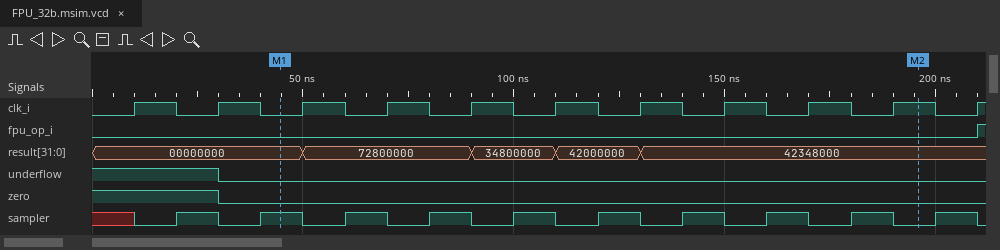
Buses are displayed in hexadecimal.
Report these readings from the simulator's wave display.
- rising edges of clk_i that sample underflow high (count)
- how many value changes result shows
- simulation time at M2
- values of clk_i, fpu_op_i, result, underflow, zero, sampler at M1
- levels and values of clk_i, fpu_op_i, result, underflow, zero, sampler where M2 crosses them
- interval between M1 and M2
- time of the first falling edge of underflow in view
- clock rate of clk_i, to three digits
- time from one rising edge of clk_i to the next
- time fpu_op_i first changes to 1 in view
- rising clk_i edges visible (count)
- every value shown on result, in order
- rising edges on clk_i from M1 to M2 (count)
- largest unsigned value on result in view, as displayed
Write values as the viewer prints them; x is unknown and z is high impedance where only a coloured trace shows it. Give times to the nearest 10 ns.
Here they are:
2
4
200 ns
clk_i=0, fpu_op_i=0, result=00000000, underflow=0, zero=0, sampler=1
clk_i=1, fpu_op_i=0, result=42348000, underflow=0, zero=0, sampler=0
150 ns
30 ns
50.0 MHz
20 ns
210 ns
11
00000000, 72800000, 34800000, 42000000, 42348000
8
72800000
